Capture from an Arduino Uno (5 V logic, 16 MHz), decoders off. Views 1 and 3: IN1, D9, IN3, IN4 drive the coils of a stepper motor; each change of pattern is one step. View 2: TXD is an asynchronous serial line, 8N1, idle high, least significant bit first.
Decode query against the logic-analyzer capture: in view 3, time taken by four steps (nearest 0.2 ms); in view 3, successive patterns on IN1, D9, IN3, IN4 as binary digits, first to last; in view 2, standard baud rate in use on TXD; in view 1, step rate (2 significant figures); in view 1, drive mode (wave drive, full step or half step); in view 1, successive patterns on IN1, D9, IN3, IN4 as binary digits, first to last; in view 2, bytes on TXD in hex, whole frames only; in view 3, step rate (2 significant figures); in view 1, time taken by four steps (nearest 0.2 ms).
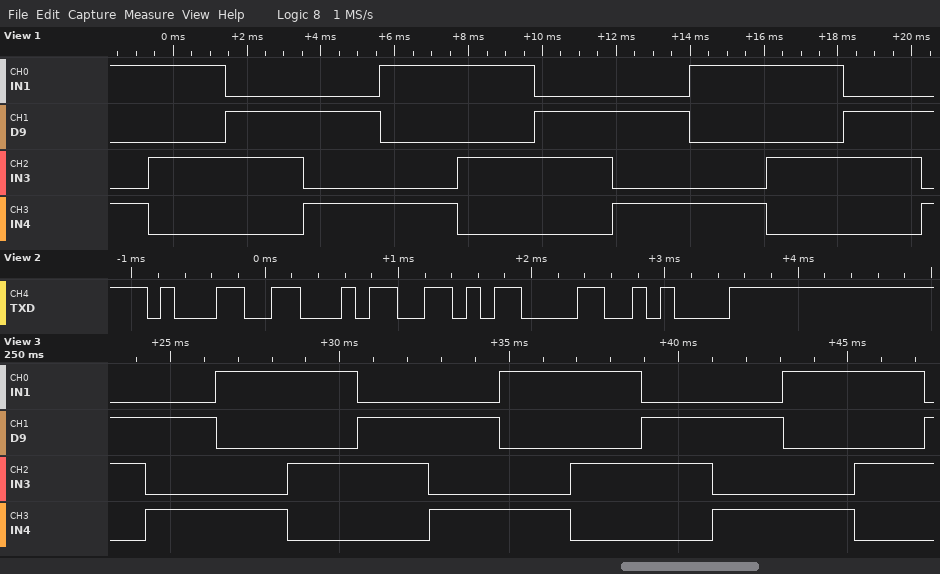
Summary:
8.4 ms
0110 0101 1001 1010 0110 0101 1001 1010 0110 0101 1001 1010 0110
9600 baud
480 steps/s
full step
1001 1010 0110 0101 1001 1010 0110 0101 1001 1010 0110 0101
31 34 0D 0A
480 steps/s
8.4 ms
